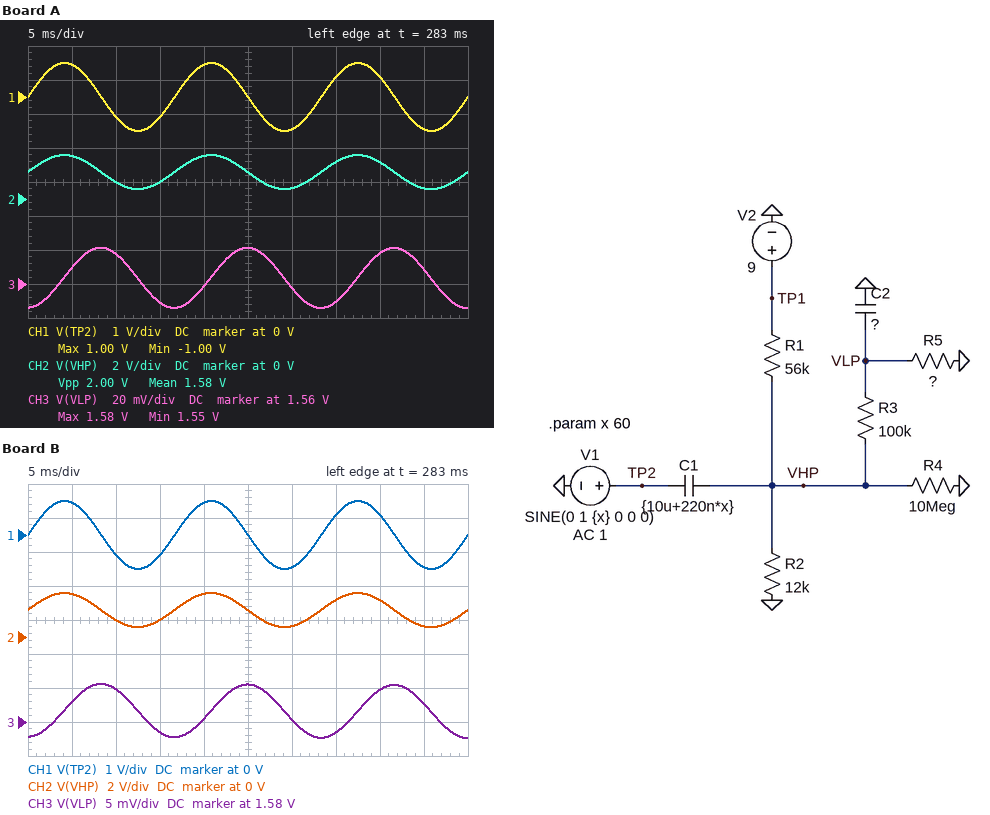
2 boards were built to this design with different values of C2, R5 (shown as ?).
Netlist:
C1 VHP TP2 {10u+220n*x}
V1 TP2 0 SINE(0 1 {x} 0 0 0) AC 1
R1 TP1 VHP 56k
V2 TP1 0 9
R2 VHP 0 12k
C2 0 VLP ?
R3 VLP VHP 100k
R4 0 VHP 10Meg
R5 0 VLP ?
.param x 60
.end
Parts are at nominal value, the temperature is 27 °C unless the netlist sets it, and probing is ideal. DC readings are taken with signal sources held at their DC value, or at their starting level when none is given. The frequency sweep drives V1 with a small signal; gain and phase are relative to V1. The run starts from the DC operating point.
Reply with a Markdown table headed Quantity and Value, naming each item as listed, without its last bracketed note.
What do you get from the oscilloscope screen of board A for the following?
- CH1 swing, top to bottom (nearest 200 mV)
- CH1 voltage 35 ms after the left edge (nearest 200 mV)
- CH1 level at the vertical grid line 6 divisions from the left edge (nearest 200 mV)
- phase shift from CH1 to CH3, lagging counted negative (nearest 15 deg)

| Quantity | Value |
|---|---|
| CH1 swing, top to bottom | 2.0 V |
| CH1 voltage 35 ms after the left edge | 600 mV |
| CH1 level at the vertical grid line 6 divisions from the left edge | -1.0 V |
| phase shift from CH1 to CH3, lagging counted negative | -90 deg |
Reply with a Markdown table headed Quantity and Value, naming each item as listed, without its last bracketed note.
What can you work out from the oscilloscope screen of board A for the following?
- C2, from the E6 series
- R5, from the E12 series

| Quantity | Value |
|---|---|
| C2, from the E6 series | 1.5 µF |
| R5, from the E12 series | 8.2 MΩ |
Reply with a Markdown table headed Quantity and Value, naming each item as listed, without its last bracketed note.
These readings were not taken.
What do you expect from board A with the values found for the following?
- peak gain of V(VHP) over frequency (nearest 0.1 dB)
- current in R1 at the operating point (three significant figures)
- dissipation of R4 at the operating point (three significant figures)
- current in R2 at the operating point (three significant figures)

| Quantity | Value |
|---|---|
| peak gain of V(VHP) over frequency | 0 dB |
| current in R1 at the operating point | 132 µA |
| dissipation of R4 at the operating point | 251 nW |
| current in R2 at the operating point | 132 µA |
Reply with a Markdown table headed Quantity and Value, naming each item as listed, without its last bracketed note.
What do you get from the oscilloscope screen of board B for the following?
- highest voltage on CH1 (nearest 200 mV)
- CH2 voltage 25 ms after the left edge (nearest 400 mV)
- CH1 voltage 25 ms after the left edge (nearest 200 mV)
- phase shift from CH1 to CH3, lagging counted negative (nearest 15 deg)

| Quantity | Value |
|---|---|
| highest voltage on CH1 | 1.0 V |
| CH2 voltage 25 ms after the left edge | 1.6 V |
| CH1 voltage 25 ms after the left edge | 0 V |
| phase shift from CH1 to CH3, lagging counted negative | -90 deg |
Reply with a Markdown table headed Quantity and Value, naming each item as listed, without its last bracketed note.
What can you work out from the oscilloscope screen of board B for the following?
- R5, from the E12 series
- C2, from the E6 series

| Quantity | Value |
|---|---|
| R5, from the E12 series | 33 MΩ |
| C2, from the E6 series | 6.8 µF |
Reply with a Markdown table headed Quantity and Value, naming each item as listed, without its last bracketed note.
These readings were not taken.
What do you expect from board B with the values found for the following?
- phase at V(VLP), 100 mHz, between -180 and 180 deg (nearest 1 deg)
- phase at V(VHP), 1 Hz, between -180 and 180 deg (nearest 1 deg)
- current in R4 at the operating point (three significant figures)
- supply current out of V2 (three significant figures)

| Quantity | Value |
|---|---|
| phase at V(VLP), 100 mHz, between -180 and 180 deg | 57 deg |
| phase at V(VHP), 1 Hz, between -180 and 180 deg | 37 deg |
| current in R4 at the operating point | 159 nA |
| supply current out of V2 | 132 µA |
